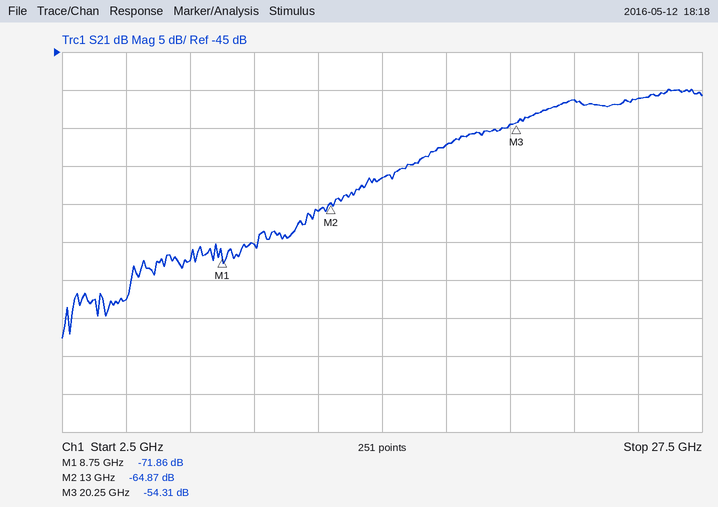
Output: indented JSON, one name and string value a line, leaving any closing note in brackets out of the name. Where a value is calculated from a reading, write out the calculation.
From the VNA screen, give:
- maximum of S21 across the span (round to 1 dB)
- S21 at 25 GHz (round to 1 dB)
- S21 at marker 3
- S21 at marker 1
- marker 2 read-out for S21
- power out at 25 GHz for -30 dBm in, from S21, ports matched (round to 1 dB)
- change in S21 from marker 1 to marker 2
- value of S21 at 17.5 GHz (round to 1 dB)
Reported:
{
  "maximum of S21 across the span": "-50 dB",
  "S21 at 25 GHz": "-51 dB",
  "S21 at marker 3": "-54.31 dB",
  "S21 at marker 1": "-71.86 dB",
  "marker 2 read-out for S21": "-64.87 dB",
  "power out at 25 GHz for -30 dBm in, from S21, ports matched": "-30 dBm + (-51 dB) = -81 dBm",
  "change in S21 from marker 1 to marker 2": "-64.87 − (-71.86) = 6.99 dB",
  "value of S21 at 17.5 GHz": "-57 dB"
}
